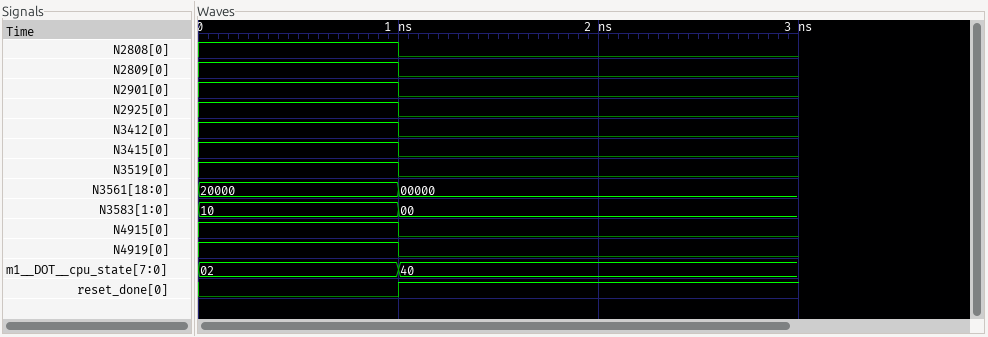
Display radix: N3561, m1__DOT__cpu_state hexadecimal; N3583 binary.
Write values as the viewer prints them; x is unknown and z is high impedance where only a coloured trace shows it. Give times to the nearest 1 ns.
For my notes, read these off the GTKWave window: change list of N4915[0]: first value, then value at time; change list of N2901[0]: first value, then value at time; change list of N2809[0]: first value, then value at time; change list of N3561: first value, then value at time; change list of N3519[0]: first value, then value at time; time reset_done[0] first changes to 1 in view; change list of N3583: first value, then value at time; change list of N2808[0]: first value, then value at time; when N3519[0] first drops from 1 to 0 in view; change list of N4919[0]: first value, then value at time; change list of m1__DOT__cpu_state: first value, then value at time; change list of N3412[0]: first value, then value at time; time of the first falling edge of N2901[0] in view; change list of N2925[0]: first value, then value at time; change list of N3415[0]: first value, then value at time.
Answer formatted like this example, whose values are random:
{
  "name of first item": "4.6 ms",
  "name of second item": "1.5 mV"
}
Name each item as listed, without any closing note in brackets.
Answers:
{
  "change list of N4915[0]: first value, then value at time": "1, 0 at 1 ns",
  "change list of N2901[0]: first value, then value at time": "1, 0 at 1 ns",
  "change list of N2809[0]: first value, then value at time": "1, 0 at 1 ns",
  "change list of N3561: first value, then value at time": "20000, 00000 at 1 ns",
  "change list of N3519[0]: first value, then value at time": "1, 0 at 1 ns",
  "time reset_done[0] first changes to 1 in view": "1 ns",
  "change list of N3583: first value, then value at time": "10, 00 at 1 ns",
  "change list of N2808[0]: first value, then value at time": "1, 0 at 1 ns",
  "when N3519[0] first drops from 1 to 0 in view": "1 ns",
  "change list of N4919[0]: first value, then value at time": "1, 0 at 1 ns",
  "change list of m1__DOT__cpu_state: first value, then value at time": "02, 40 at 1 ns",
  "change list of N3412[0]: first value, then value at time": "1, 0 at 1 ns",
  "time of the first falling edge of N2901[0] in view": "1 ns",
  "change list of N2925[0]: first value, then value at time": "1, 0 at 1 ns",
  "change list of N3415[0]: first value, then value at time": "1, 0 at 1 ns"
}
